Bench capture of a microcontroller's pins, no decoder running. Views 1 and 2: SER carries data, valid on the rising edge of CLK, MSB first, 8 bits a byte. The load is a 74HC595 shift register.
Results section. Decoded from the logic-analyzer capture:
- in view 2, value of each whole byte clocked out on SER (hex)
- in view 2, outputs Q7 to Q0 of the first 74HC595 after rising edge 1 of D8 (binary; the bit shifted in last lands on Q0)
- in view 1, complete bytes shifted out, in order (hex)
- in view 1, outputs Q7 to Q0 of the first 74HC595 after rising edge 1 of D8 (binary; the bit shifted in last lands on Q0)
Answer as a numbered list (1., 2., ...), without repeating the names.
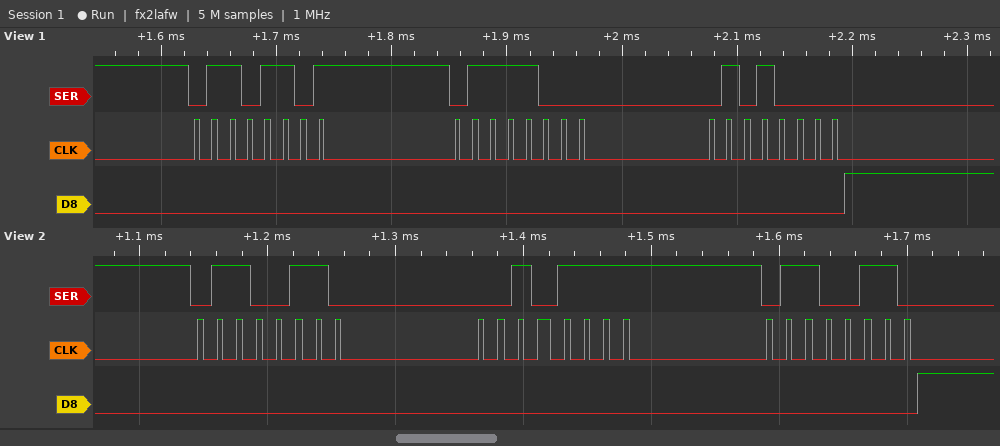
1. 66 2F 66
2. 01100110
3. 6D 78 50
4. 01010000
